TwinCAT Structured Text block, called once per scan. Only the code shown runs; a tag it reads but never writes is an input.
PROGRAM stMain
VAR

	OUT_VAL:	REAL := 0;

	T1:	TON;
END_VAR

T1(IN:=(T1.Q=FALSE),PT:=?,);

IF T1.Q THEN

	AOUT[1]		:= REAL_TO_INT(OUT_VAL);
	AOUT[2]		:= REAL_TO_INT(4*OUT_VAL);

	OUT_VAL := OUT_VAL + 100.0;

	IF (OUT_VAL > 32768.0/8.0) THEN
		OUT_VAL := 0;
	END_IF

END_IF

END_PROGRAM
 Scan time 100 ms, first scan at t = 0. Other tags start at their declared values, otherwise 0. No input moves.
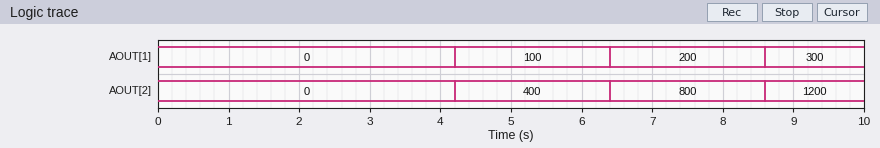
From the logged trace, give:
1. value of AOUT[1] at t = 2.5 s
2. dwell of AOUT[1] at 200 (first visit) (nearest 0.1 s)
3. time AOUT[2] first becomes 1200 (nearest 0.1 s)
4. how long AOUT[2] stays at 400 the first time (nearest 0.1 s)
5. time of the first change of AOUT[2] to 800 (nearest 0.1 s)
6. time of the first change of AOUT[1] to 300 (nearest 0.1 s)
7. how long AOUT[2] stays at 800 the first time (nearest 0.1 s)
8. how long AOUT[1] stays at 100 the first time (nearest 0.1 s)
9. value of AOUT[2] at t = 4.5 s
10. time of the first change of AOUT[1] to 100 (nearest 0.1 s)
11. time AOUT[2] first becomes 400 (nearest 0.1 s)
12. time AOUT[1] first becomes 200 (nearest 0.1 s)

0
2.2 s
8.6 s
2.2 s
6.4 s
8.6 s
2.2 s
2.2 s
400
4.2 s
4.2 s
6.4 s
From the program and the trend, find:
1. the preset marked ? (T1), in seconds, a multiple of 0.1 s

2.0 s
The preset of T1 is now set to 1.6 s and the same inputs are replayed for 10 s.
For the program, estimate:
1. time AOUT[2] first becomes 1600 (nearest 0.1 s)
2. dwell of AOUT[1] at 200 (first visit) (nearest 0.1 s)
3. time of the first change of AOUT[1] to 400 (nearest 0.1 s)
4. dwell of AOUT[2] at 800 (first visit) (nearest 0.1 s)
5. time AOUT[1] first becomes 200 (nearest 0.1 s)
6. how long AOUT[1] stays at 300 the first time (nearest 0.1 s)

8.8 s
1.8 s
8.8 s
1.8 s
5.2 s
1.8 s
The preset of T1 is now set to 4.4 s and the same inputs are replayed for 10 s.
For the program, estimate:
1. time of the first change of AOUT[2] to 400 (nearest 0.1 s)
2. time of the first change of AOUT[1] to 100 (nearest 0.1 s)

9.0 s
9.0 s
